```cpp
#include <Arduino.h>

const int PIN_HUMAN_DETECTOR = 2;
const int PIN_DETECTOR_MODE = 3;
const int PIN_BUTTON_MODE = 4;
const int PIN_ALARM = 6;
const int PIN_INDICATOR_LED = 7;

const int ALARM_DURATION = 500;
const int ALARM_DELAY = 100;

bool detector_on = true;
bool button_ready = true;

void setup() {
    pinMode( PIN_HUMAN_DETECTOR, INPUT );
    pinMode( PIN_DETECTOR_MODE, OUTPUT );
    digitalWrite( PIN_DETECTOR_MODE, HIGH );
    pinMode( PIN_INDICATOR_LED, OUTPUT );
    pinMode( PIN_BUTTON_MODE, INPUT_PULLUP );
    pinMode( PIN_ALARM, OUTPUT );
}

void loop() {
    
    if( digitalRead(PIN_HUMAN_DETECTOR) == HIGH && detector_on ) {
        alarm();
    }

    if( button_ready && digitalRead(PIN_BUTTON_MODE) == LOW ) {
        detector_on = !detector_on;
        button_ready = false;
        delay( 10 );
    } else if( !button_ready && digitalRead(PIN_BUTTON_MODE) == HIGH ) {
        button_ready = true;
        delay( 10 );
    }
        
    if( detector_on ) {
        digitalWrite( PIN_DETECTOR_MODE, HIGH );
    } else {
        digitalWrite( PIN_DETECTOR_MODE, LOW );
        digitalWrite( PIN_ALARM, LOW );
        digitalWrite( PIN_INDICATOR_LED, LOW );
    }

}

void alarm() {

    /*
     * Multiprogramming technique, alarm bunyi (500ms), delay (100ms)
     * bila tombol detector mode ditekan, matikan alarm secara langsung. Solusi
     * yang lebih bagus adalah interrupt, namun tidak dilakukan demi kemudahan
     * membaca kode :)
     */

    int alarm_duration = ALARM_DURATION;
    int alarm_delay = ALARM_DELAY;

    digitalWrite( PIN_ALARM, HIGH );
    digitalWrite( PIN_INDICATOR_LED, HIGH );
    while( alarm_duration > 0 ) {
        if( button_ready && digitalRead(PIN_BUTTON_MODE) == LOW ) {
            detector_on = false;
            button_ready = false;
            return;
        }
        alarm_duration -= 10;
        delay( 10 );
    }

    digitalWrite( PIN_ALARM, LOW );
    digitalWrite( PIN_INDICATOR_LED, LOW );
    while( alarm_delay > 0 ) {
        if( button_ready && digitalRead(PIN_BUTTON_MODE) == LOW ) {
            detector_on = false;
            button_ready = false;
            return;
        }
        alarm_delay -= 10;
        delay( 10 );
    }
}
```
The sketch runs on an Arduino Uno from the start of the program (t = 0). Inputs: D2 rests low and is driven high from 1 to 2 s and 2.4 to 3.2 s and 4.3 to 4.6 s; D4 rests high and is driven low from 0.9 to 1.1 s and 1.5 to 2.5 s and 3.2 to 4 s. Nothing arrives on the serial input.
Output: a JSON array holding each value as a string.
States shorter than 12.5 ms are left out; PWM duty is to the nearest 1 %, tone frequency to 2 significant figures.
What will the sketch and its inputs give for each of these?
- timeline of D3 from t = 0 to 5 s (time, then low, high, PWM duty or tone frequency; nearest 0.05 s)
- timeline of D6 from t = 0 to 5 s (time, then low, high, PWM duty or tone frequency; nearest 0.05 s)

["0 s high; 0.9 s low; 1.5 s high; 3.2 s low", "0 s low; 1.5 s high; 2 s low; 2.4 s high; 2.9 s low; 3 s high; 3.2 s low"]
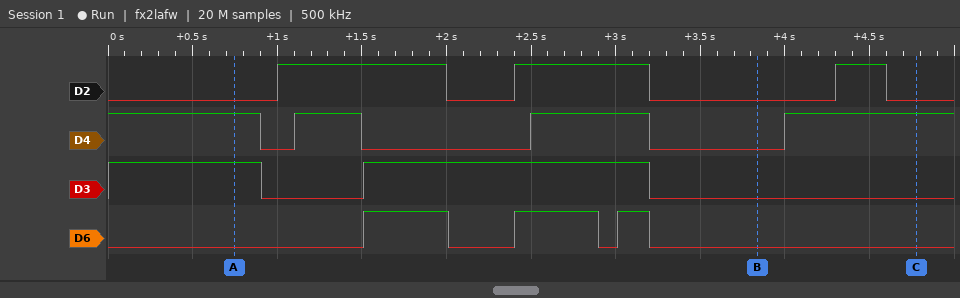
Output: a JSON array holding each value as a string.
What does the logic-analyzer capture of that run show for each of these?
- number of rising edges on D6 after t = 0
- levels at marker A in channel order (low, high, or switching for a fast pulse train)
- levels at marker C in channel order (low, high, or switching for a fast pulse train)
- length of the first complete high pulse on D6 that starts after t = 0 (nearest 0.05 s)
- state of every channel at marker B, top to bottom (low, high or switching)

["3", "D2 low, D4 high, D3 high, D6 low", "D2 low, D4 high, D3 low, D6 low", "0.50 s", "D2 low, D4 low, D3 low, D6 low"]
